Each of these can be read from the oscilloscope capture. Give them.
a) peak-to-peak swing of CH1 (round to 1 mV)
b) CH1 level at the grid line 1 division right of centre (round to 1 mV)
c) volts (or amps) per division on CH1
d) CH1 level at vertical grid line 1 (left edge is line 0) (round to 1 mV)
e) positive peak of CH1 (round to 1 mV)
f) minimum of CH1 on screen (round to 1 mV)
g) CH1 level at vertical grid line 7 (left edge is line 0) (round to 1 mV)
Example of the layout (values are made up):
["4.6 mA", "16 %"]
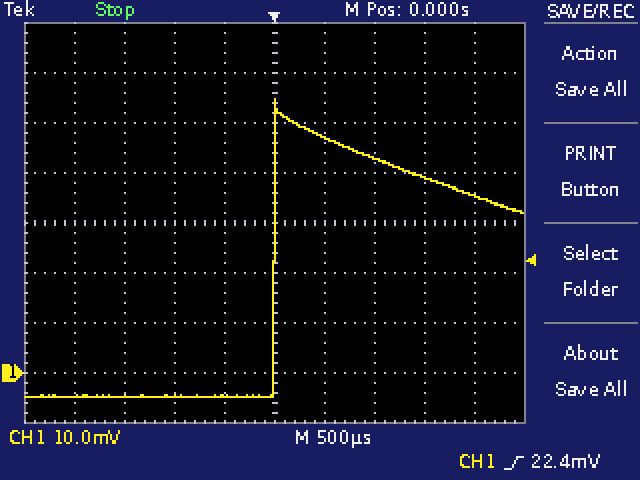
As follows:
["60 mV", "47 mV", "10 mV", "-5 mV", "55 mV", "-5 mV", "43 mV"]
